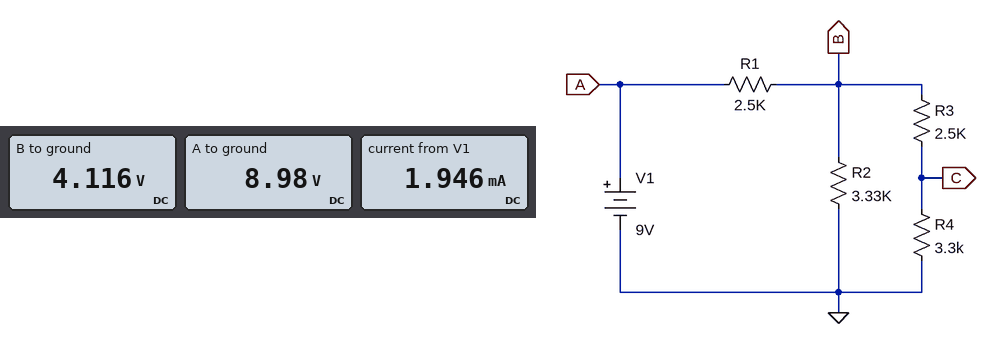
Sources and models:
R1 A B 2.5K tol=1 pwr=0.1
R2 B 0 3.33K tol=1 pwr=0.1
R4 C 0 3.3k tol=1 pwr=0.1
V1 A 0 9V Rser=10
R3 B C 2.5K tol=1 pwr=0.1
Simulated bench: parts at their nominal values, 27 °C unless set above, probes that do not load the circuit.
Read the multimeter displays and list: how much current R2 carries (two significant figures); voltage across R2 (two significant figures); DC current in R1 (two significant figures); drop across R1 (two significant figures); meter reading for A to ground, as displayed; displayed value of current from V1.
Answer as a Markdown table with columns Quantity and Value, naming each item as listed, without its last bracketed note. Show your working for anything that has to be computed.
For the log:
| Quantity | Value |
|---|---|
| how much current R2 carries | (4.116 V) / 3.33 kΩ = 1.2 mA |
| voltage across R2 | 4.116 V = 4.1 V |
| DC current in R1 | (8.98 V - 4.116 V) / 2.5 kΩ = 1.9 mA |
| drop across R1 | 8.98 V - 4.116 V = 4.9 V |
| meter reading for A to ground, as displayed | 8.98 V |
| displayed value of current from V1 | 1.946 mA |
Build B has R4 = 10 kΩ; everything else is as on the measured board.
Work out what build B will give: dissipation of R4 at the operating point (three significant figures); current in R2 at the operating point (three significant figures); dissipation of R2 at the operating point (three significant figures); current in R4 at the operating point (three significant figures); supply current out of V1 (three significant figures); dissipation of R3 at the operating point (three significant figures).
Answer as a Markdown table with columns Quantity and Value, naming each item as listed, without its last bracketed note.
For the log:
| Quantity | Value |
|---|---|
| dissipation of R4 at the operating point | 1.36 mW |
| current in R2 at the operating point | 1.38 mA |
| dissipation of R2 at the operating point | 6.37 mW |
| current in R4 at the operating point | 368 µA |
| supply current out of V1 | 1.75 mA |
| dissipation of R3 at the operating point | 339 µW |
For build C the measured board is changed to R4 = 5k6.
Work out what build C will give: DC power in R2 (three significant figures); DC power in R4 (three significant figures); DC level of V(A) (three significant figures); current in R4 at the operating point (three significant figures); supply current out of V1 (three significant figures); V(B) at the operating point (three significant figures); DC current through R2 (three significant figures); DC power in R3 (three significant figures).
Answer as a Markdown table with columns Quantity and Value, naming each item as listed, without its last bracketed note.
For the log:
| Quantity | Value |
|---|---|
| DC power in R2 | 5.71 mW |
| DC power in R4 | 1.62 mW |
| DC level of V(A) | 8.98 V |
| current in R4 at the operating point | 538 µA |
| supply current out of V1 | 1.85 mA |
| V(B) at the operating point | 4.36 V |
| DC current through R2 | 1.31 mA |
| DC power in R3 | 725 µW |
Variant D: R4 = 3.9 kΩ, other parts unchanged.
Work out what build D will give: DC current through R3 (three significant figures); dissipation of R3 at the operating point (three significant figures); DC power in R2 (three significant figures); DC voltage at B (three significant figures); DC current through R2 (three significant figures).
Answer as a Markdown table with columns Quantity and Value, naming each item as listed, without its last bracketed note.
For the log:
| Quantity | Value |
|---|---|
| DC current through R3 | 655 µA |
| dissipation of R3 at the operating point | 1.07 mW |
| DC power in R2 | 5.28 mW |
| DC voltage at B | 4.19 V |
| DC current through R2 | 1.26 mA |
